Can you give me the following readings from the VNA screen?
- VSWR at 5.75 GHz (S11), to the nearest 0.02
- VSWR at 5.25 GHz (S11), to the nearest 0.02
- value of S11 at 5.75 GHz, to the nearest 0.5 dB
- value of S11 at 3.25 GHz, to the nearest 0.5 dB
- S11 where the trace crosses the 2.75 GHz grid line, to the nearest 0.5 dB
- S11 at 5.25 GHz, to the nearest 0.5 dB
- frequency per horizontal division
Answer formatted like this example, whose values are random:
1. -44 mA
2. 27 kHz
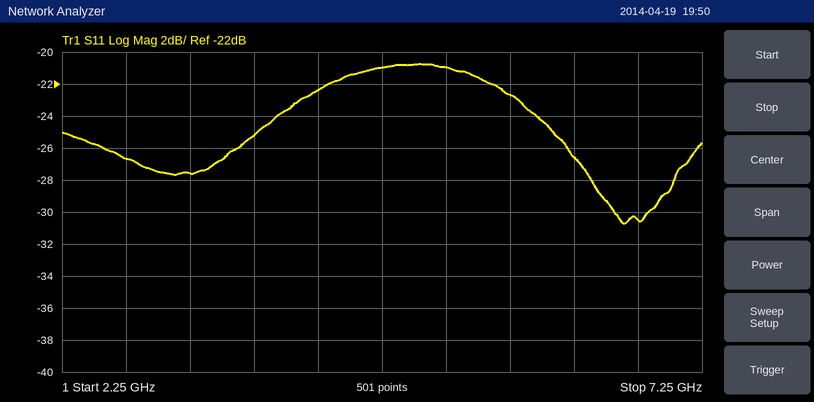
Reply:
1. 1.16
2. 1.20
3. -22.5 dB
4. -27.5 dB
5. -26.5 dB
6. -21.0 dB
7. 500 MHz
